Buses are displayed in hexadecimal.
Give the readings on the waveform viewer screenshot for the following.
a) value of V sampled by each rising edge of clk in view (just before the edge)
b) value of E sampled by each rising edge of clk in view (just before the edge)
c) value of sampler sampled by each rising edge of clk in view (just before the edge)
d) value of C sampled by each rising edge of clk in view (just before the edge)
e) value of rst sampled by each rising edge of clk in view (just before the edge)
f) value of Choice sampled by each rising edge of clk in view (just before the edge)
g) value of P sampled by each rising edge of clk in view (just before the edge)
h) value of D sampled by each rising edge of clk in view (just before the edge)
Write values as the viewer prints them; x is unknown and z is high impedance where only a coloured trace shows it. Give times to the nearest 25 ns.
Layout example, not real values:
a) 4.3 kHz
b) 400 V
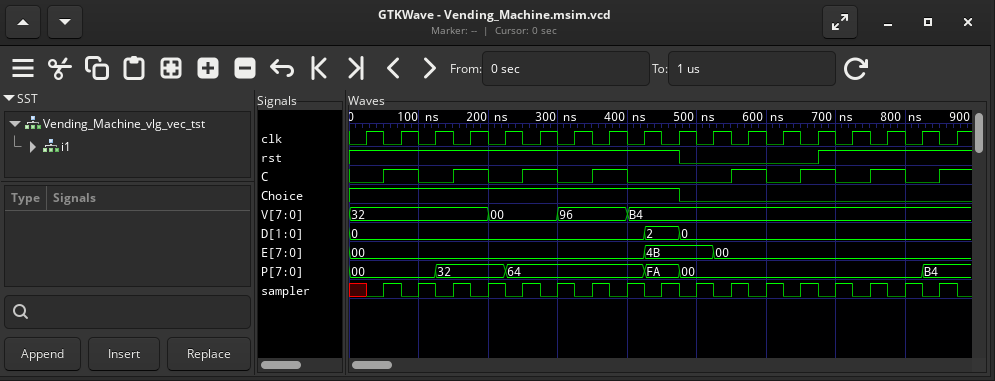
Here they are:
a) 32, 32, 32, 32, 00, 00, 96, 96, B4, B4, B4, B4, B4, B4, B4, B4, B4, B4
b) 00, 00, 00, 00, 00, 00, 00, 00, 00, 4B, 4B, 00, 00, 00, 00, 00, 00, 00
c) x 1 1 1 1 1 1 1 1 1 1 1 1 1 1 1 1 1
d) 0 1 0 1 0 1 0 1 0 0 0 1 0 1 0 1 0 1
e) 1 1 1 1 1 1 1 1 1 1 0 0 0 0 1 1 1 1
f) 1 1 1 1 1 1 1 1 1 1 0 0 0 0 0 0 0 0
g) 00, 00, 00, 32, 32, 64, 64, 64, 64, FA, 00, 00, 00, 00, 00, 00, 00, B4
h) 0, 0, 0, 0, 0, 0, 0, 0, 0, 2, 0, 0, 0, 0, 0, 0, 0, 0
